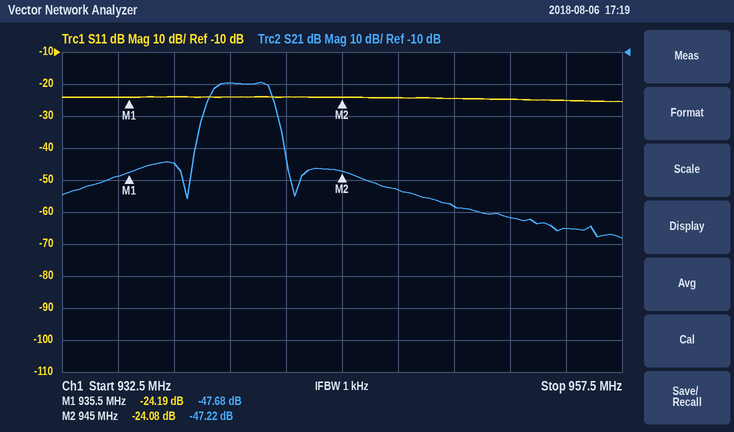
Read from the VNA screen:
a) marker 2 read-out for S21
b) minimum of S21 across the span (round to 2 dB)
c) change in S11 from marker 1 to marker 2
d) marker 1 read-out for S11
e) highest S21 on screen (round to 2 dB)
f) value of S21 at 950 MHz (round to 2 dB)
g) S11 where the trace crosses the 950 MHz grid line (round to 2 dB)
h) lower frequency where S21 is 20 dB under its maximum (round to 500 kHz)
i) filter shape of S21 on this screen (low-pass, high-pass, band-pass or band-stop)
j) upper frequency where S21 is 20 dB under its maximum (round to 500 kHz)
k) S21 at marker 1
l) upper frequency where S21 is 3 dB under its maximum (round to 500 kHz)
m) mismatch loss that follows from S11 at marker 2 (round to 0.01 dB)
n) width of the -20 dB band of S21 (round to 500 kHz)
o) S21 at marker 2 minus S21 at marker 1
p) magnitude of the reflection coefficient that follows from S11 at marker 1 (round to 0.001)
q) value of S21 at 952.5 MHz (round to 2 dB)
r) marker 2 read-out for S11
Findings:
-47.22 dB
-68 dB
0.11 dB
-24.19 dB
-20 dB
-58 dB
-24 dB
938.5 MHz
band-pass
942.5 MHz
-47.68 dB
942.0 MHz
0.02 dB
4.0 MHz
0.46 dB
0.062
-62 dB
-24.08 dB
